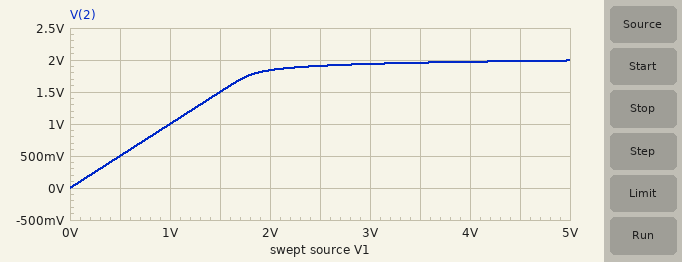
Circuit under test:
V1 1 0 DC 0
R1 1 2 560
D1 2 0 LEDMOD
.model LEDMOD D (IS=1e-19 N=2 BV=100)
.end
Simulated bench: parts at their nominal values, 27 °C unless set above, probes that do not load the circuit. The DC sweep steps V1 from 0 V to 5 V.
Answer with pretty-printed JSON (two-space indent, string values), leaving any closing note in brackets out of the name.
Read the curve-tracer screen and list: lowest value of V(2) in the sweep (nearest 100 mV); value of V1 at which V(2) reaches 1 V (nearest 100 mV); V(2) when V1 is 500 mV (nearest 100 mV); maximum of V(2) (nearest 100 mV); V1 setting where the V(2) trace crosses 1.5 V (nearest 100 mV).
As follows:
{
  "lowest value of V(2) in the sweep": "0 V",
  "value of V1 at which V(2) reaches 1 V": "1.0 V",
  "V(2) when V1 is 500 mV": "500 mV",
  "maximum of V(2)": "2.0 V",
  "V1 setting where the V(2) trace crosses 1.5 V": "1.5 V"
}
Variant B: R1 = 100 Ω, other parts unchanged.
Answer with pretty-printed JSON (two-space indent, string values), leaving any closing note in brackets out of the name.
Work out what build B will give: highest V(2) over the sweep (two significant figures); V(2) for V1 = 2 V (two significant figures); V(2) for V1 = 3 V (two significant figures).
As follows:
{
  "highest V(2) over the sweep": "2.1 V",
  "V(2) for V1 = 2 V": "1.9 V",
  "V(2) for V1 = 3 V": "2.0 V"
}
